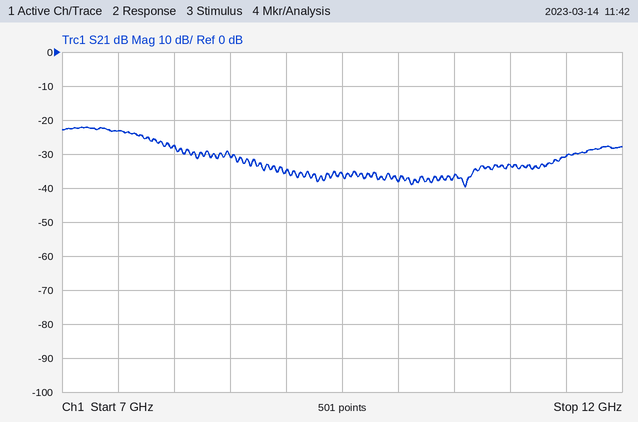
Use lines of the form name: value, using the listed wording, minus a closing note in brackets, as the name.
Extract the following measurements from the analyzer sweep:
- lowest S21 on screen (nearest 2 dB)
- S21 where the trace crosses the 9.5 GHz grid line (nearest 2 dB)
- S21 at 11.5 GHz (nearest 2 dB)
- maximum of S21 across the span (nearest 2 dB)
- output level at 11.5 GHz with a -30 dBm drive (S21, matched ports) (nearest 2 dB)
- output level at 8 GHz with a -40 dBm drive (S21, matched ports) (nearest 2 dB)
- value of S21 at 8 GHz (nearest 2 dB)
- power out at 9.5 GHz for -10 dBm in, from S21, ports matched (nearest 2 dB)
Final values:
lowest S21 on screen: -40 dB
S21 where the trace crosses the 9.5 GHz grid line: -36 dB
S21 at 11.5 GHz: -30 dB
maximum of S21 across the span: -22 dB
output level at 11.5 GHz with a -30 dBm drive (S21, matched ports): -60 dBm
output level at 8 GHz with a -40 dBm drive (S21, matched ports): -68 dBm
value of S21 at 8 GHz: -28 dB
power out at 9.5 GHz for -10 dBm in, from S21, ports matched: -46 dBm
